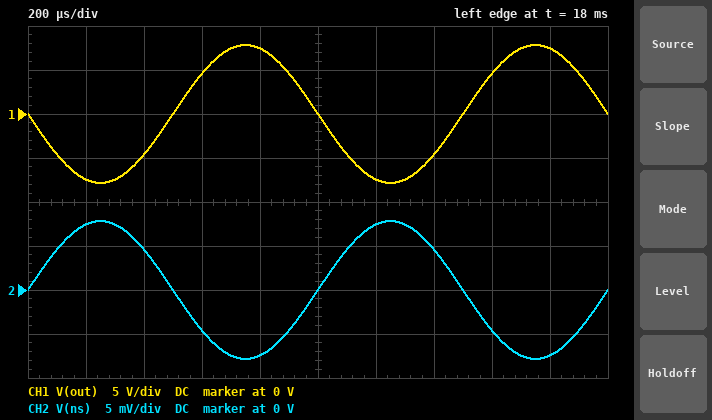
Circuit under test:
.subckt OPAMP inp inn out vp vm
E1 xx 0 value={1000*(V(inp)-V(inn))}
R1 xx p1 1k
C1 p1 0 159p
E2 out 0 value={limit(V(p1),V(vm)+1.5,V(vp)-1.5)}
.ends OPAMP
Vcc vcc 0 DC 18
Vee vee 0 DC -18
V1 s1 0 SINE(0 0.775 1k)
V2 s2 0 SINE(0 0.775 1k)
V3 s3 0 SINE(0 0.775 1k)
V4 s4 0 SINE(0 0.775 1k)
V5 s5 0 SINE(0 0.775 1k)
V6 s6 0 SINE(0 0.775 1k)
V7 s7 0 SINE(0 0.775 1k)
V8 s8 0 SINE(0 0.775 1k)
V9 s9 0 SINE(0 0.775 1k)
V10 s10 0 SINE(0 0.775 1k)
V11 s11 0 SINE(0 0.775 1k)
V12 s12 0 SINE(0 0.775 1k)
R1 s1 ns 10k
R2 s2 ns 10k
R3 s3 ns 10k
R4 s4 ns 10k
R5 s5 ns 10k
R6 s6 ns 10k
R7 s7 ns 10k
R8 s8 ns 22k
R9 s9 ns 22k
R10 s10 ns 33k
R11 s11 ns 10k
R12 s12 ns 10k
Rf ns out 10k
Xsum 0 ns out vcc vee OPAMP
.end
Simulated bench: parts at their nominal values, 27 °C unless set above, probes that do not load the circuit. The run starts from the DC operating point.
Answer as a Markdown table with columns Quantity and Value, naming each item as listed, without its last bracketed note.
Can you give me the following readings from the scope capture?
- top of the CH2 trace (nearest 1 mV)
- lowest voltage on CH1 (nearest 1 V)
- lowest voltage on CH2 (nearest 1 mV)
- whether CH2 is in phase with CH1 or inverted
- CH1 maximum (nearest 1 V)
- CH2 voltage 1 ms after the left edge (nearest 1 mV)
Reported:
| Quantity | Value |
|---|---|
| top of the CH2 trace | 8 mV |
| lowest voltage on CH1 | -8 V |
| lowest voltage on CH2 | -8 mV |
| whether CH2 is in phase with CH1 or inverted | inverted |
| CH1 maximum | 8 V |
| CH2 voltage 1 ms after the left edge | 0 V |
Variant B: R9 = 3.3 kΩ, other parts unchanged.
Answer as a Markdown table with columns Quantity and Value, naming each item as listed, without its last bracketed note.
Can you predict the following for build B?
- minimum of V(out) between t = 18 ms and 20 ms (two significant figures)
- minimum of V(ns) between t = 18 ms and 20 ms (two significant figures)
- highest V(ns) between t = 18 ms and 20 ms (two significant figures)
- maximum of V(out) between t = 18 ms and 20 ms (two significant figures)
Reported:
| Quantity | Value |
|---|---|
| minimum of V(out) between t = 18 ms and 20 ms | -9.8 V |
| minimum of V(ns) between t = 18 ms and 20 ms | -9.8 mV |
| highest V(ns) between t = 18 ms and 20 ms | 9.8 mV |
| maximum of V(out) between t = 18 ms and 20 ms | 9.8 V |
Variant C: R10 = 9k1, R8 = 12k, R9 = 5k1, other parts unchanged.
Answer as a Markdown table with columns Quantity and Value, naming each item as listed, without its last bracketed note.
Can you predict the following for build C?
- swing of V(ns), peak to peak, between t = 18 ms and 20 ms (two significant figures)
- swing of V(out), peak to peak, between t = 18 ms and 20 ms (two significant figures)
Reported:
| Quantity | Value |
|---|---|
| swing of V(ns), peak to peak, between t = 18 ms and 20 ms | 20 mV |
| swing of V(out), peak to peak, between t = 18 ms and 20 ms | 20 V |
